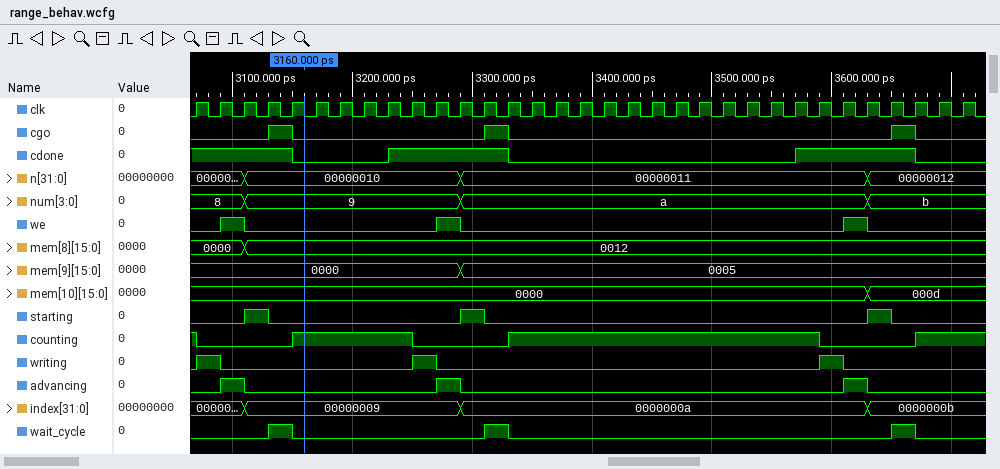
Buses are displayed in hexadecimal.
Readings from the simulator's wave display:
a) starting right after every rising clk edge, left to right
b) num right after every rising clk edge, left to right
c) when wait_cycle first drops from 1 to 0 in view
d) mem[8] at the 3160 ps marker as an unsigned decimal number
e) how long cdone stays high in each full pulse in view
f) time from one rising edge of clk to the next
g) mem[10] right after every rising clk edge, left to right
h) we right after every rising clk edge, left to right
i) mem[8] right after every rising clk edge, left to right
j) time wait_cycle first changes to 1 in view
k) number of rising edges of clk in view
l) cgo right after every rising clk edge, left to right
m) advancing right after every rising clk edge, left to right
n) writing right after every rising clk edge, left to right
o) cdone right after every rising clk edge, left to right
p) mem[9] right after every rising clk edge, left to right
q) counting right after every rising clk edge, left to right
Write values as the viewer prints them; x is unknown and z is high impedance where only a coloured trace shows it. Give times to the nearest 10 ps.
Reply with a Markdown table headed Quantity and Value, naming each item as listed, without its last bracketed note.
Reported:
| Quantity | Value |
|---|---|
| starting right after every rising clk edge, left to right | 0 0 1 0 0 0 0 0 0 0 0 1 0 0 0 0 0 0 0 0 0 0 0 0 0 0 0 0 1 0 0 0 0 |
| num right after every rising clk edge, left to right | 8, 8, 9, 9, 9, 9, 9, 9, 9, 9, 9, a, a, a, a, a, a, a, a, a, a, a, a, a, a, a, a, a, b, b, b, b, b |
| when wait_cycle first drops from 1 to 0 in view | 3150 ps |
| mem[8] at the 3160 ps marker as an unsigned decimal number | 18 |
| how long cdone stays high in each full pulse in view | 100 ps, 100 ps |
| time from one rising edge of clk to the next | 20 ps |
| mem[10] right after every rising clk edge, left to right | 0000, 0000, 0000, 0000, 0000, 0000, 0000, 0000, 0000, 0000, 0000, 0000, 0000, 0000, 0000, 0000, 0000, 0000, 0000, 0000, 0000, 0000, 0000, 0000, 0000, 0000, 0000, 0000, 000d, 000d, 000d, 000d, 000d |
| we right after every rising clk edge, left to right | 0 1 0 0 0 0 0 0 0 0 1 0 0 0 0 0 0 0 0 0 0 0 0 0 0 0 0 1 0 0 0 0 0 |
| mem[8] right after every rising clk edge, left to right | 0000, 0000, 0012, 0012, 0012, 0012, 0012, 0012, 0012, 0012, 0012, 0012, 0012, 0012, 0012, 0012, 0012, 0012, 0012, 0012, 0012, 0012, 0012, 0012, 0012, 0012, 0012, 0012, 0012, 0012, 0012, 0012, 0012 |
| time wait_cycle first changes to 1 in view | 3130 ps |
| number of rising edges of clk in view | 33 |
| cgo right after every rising clk edge, left to right | 0 0 0 1 0 0 0 0 0 0 0 0 1 0 0 0 0 0 0 0 0 0 0 0 0 0 0 0 0 1 0 0 0 |
| advancing right after every rising clk edge, left to right | 0 1 0 0 0 0 0 0 0 0 1 0 0 0 0 0 0 0 0 0 0 0 0 0 0 0 0 1 0 0 0 0 0 |
| writing right after every rising clk edge, left to right | 1 0 0 0 0 0 0 0 0 1 0 0 0 0 0 0 0 0 0 0 0 0 0 0 0 0 1 0 0 0 0 0 0 |
| cdone right after every rising clk edge, left to right | 1 1 1 1 0 0 0 0 1 1 1 1 1 0 0 0 0 0 0 0 0 0 0 0 0 1 1 1 1 1 0 0 0 |
| mem[9] right after every rising clk edge, left to right | 0000, 0000, 0000, 0000, 0000, 0000, 0000, 0000, 0000, 0000, 0000, 0005, 0005, 0005, 0005, 0005, 0005, 0005, 0005, 0005, 0005, 0005, 0005, 0005, 0005, 0005, 0005, 0005, 0005, 0005, 0005, 0005, 0005 |
| counting right after every rising clk edge, left to right | 0 0 0 0 1 1 1 1 1 0 0 0 0 1 1 1 1 1 1 1 1 1 1 1 1 1 0 0 0 0 1 1 1 |
